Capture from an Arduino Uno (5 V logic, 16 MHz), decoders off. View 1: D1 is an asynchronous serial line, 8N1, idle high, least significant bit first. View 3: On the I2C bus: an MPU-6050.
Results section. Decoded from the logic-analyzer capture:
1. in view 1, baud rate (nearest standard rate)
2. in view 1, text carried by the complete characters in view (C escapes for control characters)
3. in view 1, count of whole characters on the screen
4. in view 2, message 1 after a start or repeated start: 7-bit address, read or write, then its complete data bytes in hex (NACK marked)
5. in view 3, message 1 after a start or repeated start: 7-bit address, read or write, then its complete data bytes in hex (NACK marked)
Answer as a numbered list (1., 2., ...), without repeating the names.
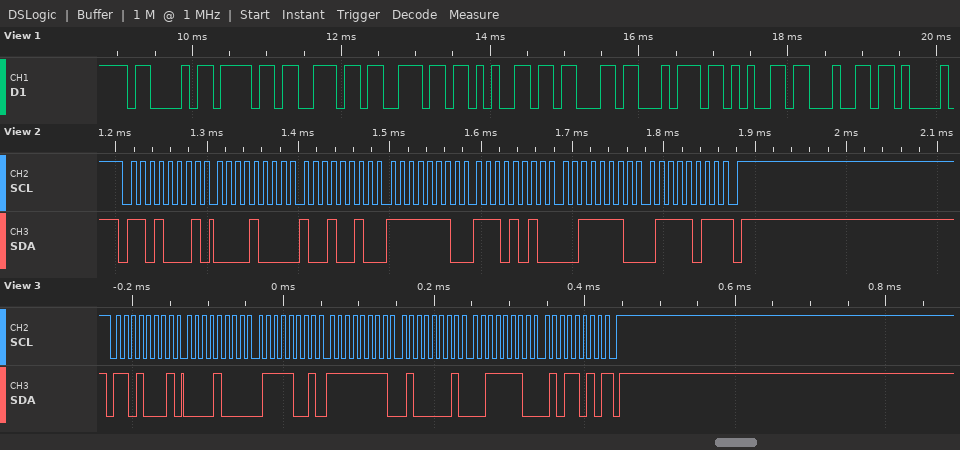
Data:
1. 9600 baud
2. "Connected"
3. 9
4. 0x68 read: 08 92 FE EA 3E 7B NACK
5. 0x68 read: 08 79 FF 41 3E 5A NACK
